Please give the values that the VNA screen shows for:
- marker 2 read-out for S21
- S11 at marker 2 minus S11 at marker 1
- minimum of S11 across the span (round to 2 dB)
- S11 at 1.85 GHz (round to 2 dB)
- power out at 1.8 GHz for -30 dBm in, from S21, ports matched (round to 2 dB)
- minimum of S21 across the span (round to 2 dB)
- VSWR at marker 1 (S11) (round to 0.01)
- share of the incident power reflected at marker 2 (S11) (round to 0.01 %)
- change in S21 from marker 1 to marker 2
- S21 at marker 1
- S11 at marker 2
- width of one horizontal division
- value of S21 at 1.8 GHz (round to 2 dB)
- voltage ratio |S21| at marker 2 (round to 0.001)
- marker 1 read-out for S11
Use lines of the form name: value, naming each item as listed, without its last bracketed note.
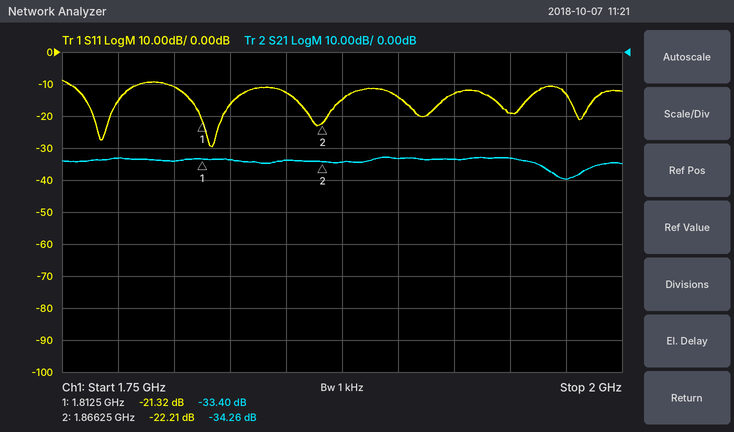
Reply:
marker 2 read-out for S21: -34.26 dB
S11 at marker 2 minus S11 at marker 1: -0.89 dB
minimum of S11 across the span: -30 dB
S11 at 1.85 GHz: -12 dB
power out at 1.8 GHz for -30 dBm in, from S21, ports matched: -64 dBm
minimum of S21 across the span: -40 dB
VSWR at marker 1 (S11): 1.19
share of the incident power reflected at marker 2 (S11): 0.60 %
change in S21 from marker 1 to marker 2: -0.86 dB
S21 at marker 1: -33.40 dB
S11 at marker 2: -22.21 dB
width of one horizontal division: 25 MHz
value of S21 at 1.8 GHz: -34 dB
voltage ratio |S21| at marker 2: 0.019
marker 1 read-out for S11: -21.32 dB
